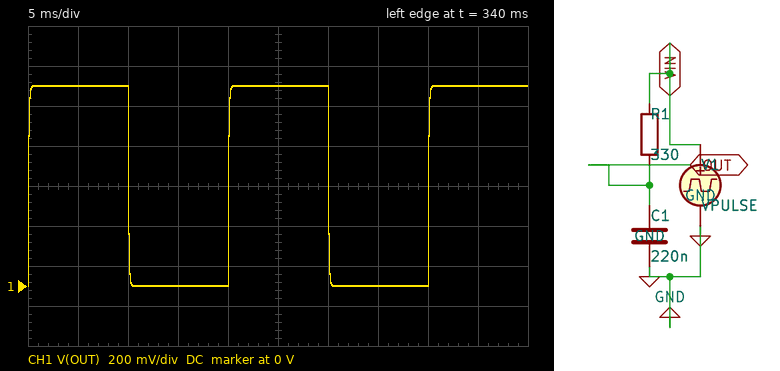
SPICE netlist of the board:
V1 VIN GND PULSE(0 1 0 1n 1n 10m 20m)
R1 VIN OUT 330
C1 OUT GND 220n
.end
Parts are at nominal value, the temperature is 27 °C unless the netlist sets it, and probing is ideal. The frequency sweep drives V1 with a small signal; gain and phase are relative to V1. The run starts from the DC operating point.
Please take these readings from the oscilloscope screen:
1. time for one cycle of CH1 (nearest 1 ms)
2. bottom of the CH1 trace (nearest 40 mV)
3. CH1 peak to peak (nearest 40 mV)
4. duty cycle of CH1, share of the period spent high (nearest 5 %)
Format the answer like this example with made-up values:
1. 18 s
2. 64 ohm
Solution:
1. 20 ms
2. 0 V
3. 1.00 V
4. 50 %
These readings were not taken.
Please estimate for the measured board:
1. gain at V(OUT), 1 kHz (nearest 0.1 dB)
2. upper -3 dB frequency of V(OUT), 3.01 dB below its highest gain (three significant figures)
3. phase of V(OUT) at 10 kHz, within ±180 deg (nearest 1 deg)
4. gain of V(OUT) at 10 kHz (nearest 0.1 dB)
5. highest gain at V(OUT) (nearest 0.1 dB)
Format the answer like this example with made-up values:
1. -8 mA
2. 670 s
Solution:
1. -0.8 dB
2. 2.19 kHz
3. -78 deg
4. -13.4 dB
5. 0 dB
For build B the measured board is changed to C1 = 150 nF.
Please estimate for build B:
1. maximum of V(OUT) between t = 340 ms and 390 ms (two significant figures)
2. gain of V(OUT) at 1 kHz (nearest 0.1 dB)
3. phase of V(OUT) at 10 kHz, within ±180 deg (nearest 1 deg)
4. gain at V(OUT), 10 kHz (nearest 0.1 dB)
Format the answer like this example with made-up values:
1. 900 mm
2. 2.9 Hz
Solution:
1. 1.0 V
2. -0.4 dB
3. -72 deg
4. -10.3 dB
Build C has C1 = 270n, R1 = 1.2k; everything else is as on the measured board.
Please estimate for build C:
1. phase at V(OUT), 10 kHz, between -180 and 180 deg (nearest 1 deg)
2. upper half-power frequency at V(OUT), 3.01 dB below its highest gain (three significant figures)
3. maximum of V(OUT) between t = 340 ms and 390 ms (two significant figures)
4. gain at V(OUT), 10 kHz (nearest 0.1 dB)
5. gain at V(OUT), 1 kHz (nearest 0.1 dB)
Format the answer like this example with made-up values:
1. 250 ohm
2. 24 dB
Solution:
1. -87 deg
2. 491 Hz
3. 1.0 V
4. -26.2 dB
5. -7.1 dB
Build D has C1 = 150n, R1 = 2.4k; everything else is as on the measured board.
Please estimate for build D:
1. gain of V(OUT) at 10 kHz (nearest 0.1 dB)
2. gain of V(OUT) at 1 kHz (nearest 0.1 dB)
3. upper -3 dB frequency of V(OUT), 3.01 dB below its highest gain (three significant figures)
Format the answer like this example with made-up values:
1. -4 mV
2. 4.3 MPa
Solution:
1. -27.1 dB
2. -7.9 dB
3. 442 Hz
